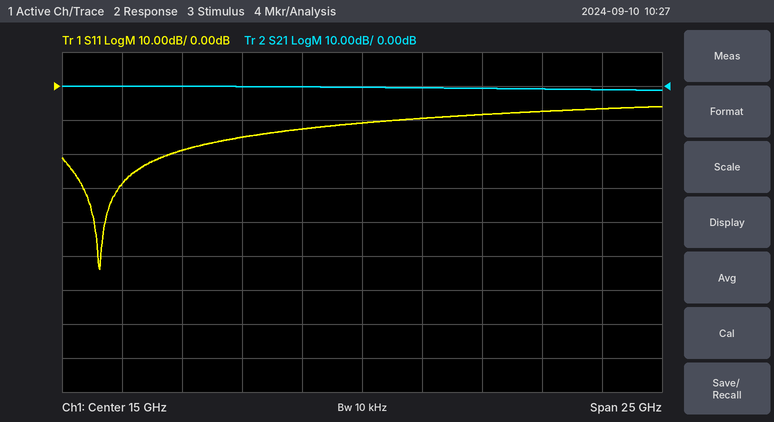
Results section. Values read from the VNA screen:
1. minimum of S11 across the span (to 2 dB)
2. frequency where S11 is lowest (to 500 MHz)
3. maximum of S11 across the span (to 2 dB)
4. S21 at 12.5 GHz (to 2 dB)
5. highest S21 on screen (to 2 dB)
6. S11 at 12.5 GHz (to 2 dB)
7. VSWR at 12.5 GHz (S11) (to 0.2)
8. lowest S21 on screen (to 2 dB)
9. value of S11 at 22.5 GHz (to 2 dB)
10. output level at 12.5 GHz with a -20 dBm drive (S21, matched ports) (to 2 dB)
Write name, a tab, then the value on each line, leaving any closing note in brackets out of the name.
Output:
minimum of S11 across the span	-54 dB
frequency where S11 is lowest	4.0 GHz
maximum of S11 across the span	-6 dB
S21 at 12.5 GHz	0 dB
highest S21 on screen	0 dB
S11 at 12.5 GHz	-12 dB
VSWR at 12.5 GHz (S11)	1.6
lowest S21 on screen	-2 dB
value of S11 at 22.5 GHz	-8 dB
output level at 12.5 GHz with a -20 dBm drive (S21, matched ports)	-20 dBm
